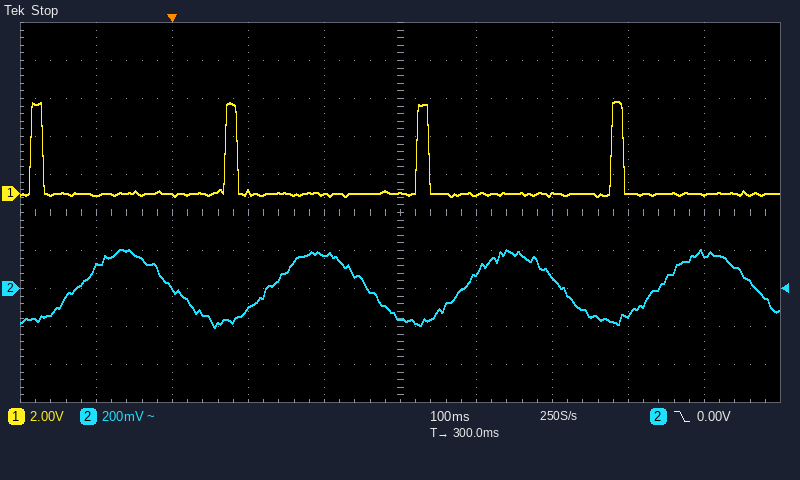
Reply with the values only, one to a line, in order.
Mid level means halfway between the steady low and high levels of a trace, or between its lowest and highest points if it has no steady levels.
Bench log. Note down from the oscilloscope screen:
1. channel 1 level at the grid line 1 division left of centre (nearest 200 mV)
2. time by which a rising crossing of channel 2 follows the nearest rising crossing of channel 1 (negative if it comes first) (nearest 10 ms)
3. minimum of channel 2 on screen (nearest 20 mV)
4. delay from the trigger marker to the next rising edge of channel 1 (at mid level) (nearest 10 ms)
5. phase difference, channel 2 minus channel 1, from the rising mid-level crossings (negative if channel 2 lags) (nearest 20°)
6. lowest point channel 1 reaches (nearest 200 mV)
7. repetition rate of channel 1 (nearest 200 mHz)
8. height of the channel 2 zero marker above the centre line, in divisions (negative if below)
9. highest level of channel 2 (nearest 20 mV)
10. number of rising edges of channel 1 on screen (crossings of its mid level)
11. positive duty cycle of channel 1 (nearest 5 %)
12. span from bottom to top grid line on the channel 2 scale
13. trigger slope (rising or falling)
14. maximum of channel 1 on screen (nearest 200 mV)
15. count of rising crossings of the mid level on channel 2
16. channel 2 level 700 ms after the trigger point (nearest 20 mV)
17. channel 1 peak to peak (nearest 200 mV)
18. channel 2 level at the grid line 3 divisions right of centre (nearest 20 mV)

0.0 V
+60 ms
-200 mV
70 ms
-80°
-200 mV
4.0 Hz
-2.0 div
200 mV
4
5 %
2 V
falling
4.8 V
4
180 mV
5.0 V
-140 mV
